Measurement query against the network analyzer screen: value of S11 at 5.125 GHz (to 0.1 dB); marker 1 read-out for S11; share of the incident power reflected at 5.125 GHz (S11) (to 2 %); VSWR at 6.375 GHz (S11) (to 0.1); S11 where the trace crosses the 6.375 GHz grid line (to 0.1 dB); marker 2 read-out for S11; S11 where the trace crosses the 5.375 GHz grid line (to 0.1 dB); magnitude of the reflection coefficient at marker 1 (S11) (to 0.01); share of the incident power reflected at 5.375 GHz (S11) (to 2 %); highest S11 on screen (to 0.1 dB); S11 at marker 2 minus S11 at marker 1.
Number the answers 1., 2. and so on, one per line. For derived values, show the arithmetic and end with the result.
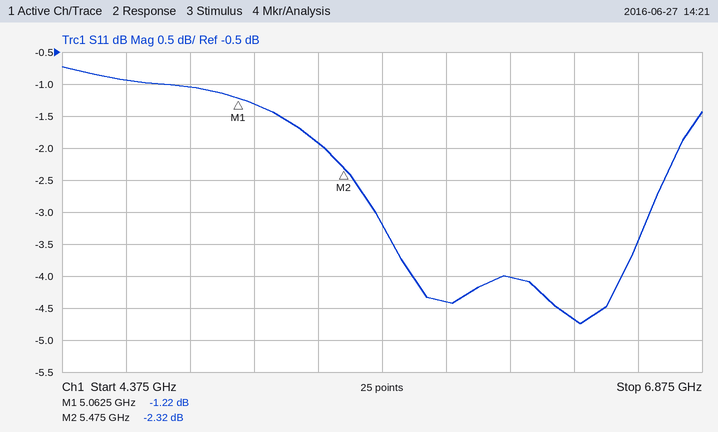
1. -1.3 dB
2. -1.22 dB
3. 10^(-1.3/10) ≈ 74 %
4. |Γ| = 10^(-4.7/20) = 0.5821; VSWR = (1 + 0.5821)/(1 − 0.5821) ≈ 3.8
5. -4.7 dB
6. -2.32 dB
7. -1.9 dB
8. 10^(-1.22/20) ≈ 0.87
9. 10^(-1.9/10) ≈ 64.6 %, so 64 % to the nearest 2 %
10. -0.7 dB
11. -2.32 − (-1.22) = -1.10 dB
